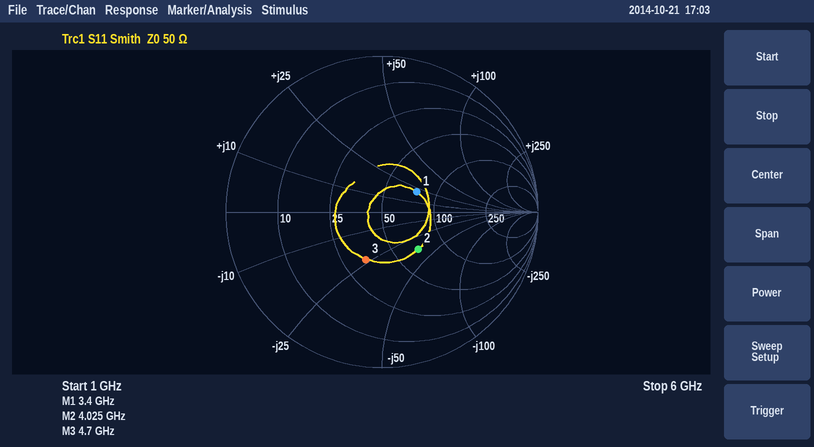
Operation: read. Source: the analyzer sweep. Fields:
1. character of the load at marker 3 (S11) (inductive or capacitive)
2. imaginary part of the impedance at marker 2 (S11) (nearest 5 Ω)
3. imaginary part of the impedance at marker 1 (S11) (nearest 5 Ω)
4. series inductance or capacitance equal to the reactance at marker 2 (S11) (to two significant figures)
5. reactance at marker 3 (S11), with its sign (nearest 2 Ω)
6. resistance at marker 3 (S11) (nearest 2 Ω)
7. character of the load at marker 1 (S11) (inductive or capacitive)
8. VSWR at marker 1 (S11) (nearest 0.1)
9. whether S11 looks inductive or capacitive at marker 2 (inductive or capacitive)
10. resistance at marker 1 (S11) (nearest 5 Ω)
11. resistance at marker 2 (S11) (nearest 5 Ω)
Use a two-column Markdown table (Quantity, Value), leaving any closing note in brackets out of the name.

| Quantity | Value |
|---|---|
| character of the load at marker 3 (S11) | capacitive |
| imaginary part of the impedance at marker 2 (S11) | -35 Ω |
| imaginary part of the impedance at marker 1 (S11) | +20 Ω |
| series inductance or capacitance equal to the reactance at marker 2 (S11) | 1.1 pF |
| reactance at marker 3 (S11), with its sign | -24 Ω |
| resistance at marker 3 (S11) | 34 Ω |
| character of the load at marker 1 (S11) | inductive |
| VSWR at marker 1 (S11) | 1.7 |
| whether S11 looks inductive or capacitive at marker 2 | capacitive |
| resistance at marker 1 (S11) | 75 Ω |
| resistance at marker 2 (S11) | 70 Ω |
